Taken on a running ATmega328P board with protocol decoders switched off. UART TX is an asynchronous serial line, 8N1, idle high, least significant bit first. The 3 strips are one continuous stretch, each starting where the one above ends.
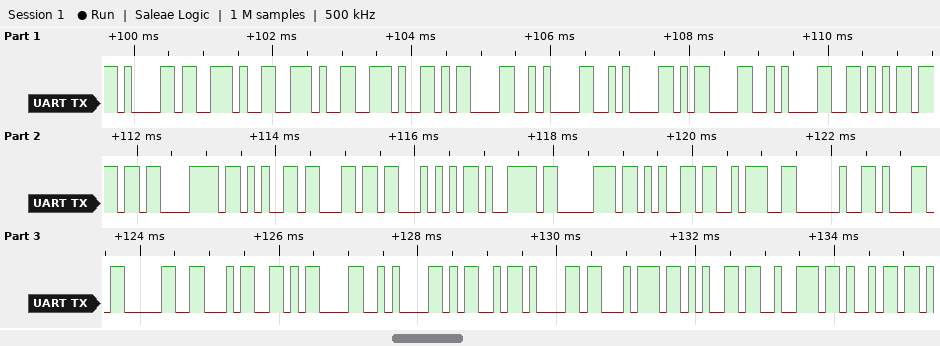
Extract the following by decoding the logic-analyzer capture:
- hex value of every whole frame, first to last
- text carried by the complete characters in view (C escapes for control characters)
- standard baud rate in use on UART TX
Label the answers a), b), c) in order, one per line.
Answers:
a) 61 2E 2E 2E 0D 0A 0A 0D 0A 56 6F 78 65 6C 54 79 70 65 3A 20 31 30 34 0D 0A 4D 61 74 65 72 69
b) "a...\r\n\n\r\nVoxelType: 104\r\nMateri"
c) 9600 baud
